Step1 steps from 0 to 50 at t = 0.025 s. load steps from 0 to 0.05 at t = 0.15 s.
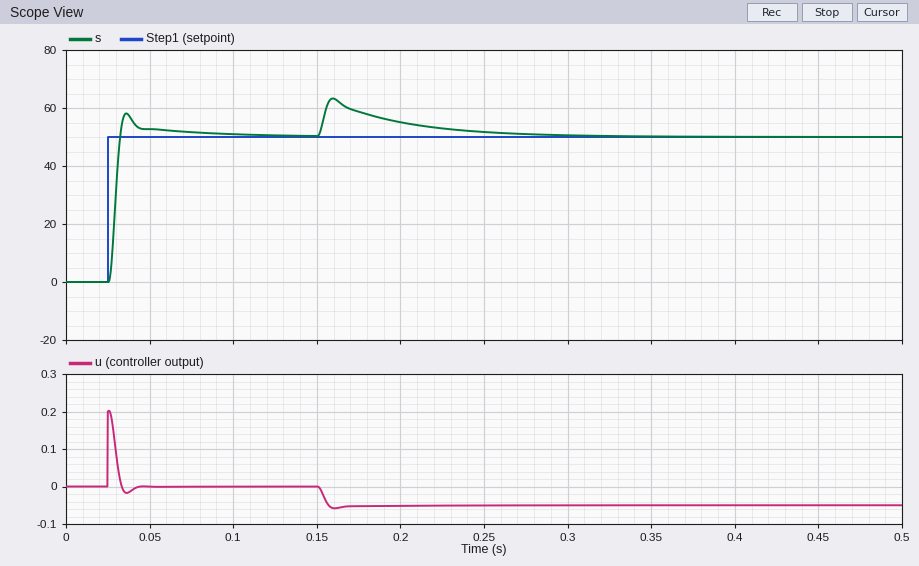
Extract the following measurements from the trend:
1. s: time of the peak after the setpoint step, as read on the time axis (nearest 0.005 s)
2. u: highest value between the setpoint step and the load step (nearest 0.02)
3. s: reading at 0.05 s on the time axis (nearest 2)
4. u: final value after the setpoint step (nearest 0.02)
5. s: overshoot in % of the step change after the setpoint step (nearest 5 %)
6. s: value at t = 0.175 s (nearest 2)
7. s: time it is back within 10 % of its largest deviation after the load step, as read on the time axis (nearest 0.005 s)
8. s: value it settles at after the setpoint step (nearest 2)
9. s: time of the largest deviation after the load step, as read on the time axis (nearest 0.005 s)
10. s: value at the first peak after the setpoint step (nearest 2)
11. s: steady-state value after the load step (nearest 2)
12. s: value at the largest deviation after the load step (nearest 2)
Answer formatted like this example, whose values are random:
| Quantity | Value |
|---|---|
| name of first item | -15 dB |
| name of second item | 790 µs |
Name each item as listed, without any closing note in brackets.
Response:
| Quantity | Value |
|---|---|
| s: time of the peak after the setpoint step, as read on the time axis | 0.035 s |
| u: highest value between the setpoint step and the load step | 0.20 |
| s: reading at 0.05 s on the time axis | 52 |
| u: final value after the setpoint step | 0.00 |
| s: overshoot in % of the step change after the setpoint step | 15 % |
| s: value at t = 0.175 s | 58 |
| s: time it is back within 10 % of its largest deviation after the load step, as read on the time axis | 0.265 s |
| s: value it settles at after the setpoint step | 50 |
| s: time of the largest deviation after the load step, as read on the time axis | 0.160 s |
| s: value at the first peak after the setpoint step | 58 |
| s: steady-state value after the load step | 50 |
| s: value at the largest deviation after the load step | 64 |
